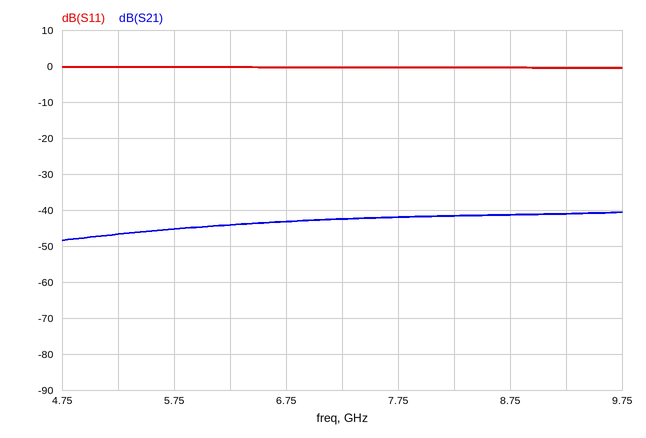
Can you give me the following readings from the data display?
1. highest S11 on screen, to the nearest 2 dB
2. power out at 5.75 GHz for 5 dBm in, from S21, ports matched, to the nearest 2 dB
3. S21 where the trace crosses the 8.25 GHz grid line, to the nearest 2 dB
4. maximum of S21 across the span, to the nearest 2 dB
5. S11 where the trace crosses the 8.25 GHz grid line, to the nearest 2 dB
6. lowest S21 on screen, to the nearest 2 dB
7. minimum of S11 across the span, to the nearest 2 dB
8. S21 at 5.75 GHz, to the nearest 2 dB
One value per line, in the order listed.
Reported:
0 dB
-40 dBm
-42 dB
-40 dB
0 dB
-48 dB
0 dB
-46 dB
